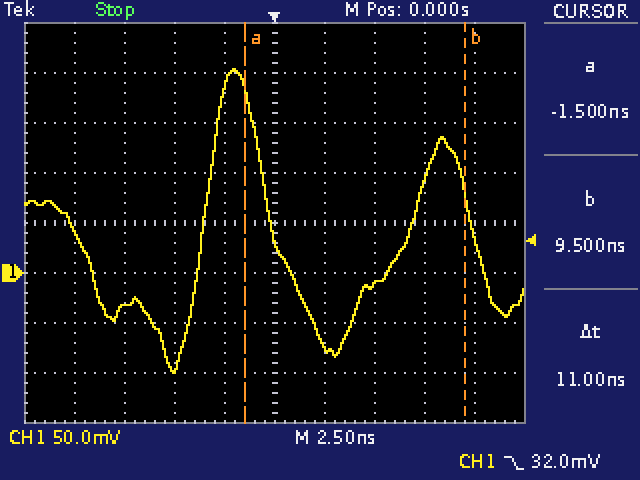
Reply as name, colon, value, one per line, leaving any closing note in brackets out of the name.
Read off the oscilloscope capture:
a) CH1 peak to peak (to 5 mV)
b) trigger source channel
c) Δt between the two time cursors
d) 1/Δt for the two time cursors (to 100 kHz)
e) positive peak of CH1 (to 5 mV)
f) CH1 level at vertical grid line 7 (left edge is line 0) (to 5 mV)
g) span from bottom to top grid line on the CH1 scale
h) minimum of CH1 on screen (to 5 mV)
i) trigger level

CH1 peak to peak: 305 mV
trigger source channel: CH1
Δt between the two time cursors: 11 ns
1/Δt for the two time cursors: 90.9 MHz
positive peak of CH1: 205 mV
CH1 level at vertical grid line 7 (left edge is line 0): -10 mV
span from bottom to top grid line on the CH1 scale: 400 mV
minimum of CH1 on screen: -100 mV
trigger level: 32.0 mV
